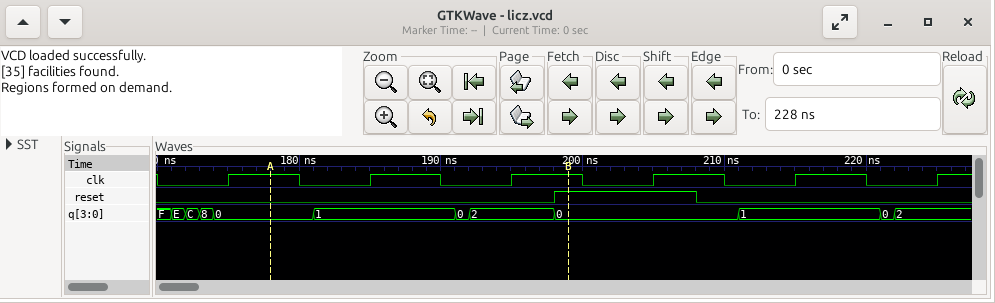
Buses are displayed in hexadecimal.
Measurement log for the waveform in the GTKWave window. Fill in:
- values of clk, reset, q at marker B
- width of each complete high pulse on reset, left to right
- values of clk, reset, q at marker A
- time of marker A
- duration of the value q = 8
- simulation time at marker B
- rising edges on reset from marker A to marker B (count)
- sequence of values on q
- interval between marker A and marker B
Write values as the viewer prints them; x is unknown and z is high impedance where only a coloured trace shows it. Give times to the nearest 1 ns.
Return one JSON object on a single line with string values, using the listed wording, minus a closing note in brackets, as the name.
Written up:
{"values of clk, reset, q at marker B": "clk=1, reset=1, q=0", "width of each complete high pulse on reset, left to right": "10 ns", "values of clk, reset, q at marker A": "clk=1, reset=0, q=0", "time of marker A": "178 ns", "duration of the value q = 8": "1 ns", "simulation time at marker B": "199 ns", "rising edges on reset from marker A to marker B": "1", "sequence of values on q": "F, E, C, 8, 0, 1, 0, 2, 0, 1, 0, 2", "interval between marker A and marker B": "21 ns"}
